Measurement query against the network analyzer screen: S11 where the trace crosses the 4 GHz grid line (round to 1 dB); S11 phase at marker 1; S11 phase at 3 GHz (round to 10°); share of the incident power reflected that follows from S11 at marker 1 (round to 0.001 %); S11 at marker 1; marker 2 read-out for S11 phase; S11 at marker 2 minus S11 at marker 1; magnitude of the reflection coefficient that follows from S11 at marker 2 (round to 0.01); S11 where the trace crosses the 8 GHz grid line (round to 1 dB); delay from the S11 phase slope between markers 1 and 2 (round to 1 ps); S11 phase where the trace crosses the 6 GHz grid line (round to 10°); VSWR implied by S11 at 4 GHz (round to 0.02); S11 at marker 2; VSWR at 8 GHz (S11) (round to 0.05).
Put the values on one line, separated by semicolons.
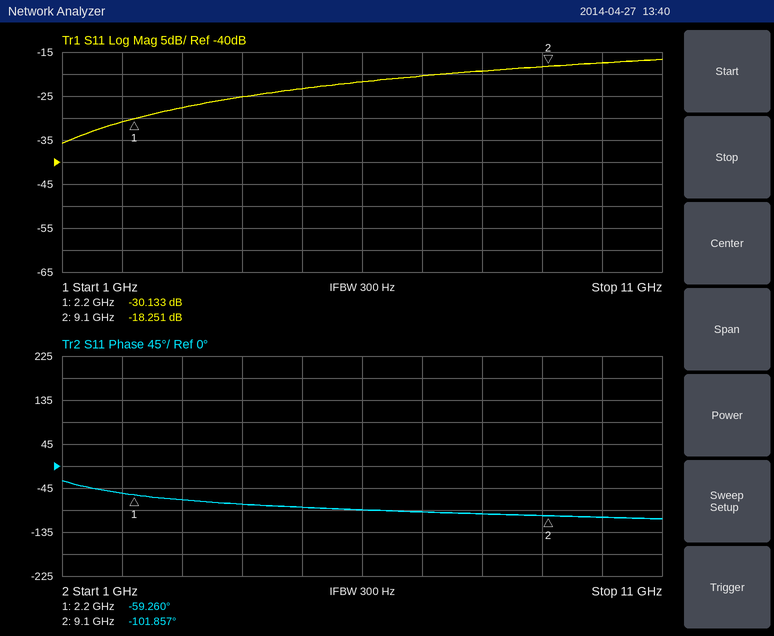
-25 dB; -59.260°; -70°; 0.097 %; -30.133 dB; -101.857°; 11.882 dB; 0.12; -19 dB; 17 ps; -90°; 1.12; -18.251 dB; 1.25
